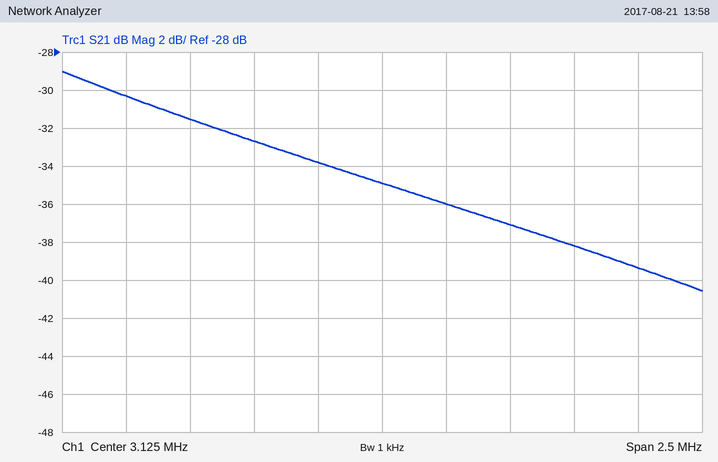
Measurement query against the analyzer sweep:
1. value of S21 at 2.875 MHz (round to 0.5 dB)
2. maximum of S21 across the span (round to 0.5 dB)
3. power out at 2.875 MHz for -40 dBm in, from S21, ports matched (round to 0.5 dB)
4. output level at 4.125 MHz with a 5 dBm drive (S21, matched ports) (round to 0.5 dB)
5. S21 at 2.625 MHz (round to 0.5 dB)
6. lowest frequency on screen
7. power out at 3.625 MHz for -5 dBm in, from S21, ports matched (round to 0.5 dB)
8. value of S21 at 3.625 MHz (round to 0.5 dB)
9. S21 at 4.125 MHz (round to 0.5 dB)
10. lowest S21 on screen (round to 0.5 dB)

-34.0 dB
-29.0 dB
-74.0 dBm
-34.5 dBm
-32.5 dB
1.875 MHz
-42.0 dBm
-37.0 dB
-39.5 dB
-40.5 dB
